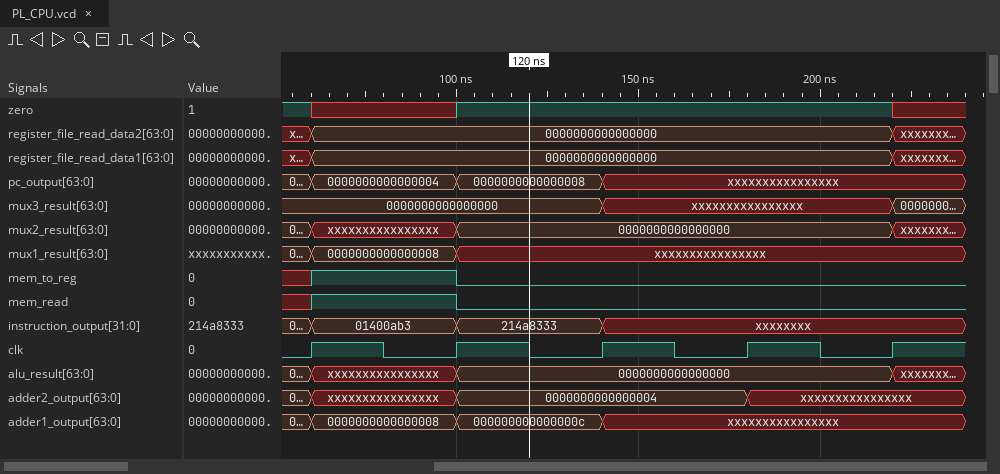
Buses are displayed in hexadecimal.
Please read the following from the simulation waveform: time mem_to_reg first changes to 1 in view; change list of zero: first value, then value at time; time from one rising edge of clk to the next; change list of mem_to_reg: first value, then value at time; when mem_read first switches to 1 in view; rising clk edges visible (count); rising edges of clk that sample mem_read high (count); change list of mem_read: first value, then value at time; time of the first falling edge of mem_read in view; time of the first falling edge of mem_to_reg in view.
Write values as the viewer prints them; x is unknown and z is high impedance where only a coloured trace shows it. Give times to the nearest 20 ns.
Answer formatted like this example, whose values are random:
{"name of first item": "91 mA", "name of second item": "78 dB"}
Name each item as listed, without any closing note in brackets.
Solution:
{"time mem_to_reg first changes to 1 in view": "60 ns", "change list of zero: first value, then value at time": "1, x at 60 ns, 1 at 100 ns, x at 220 ns", "time from one rising edge of clk to the next": "40 ns", "change list of mem_to_reg: first value, then value at time": "x, 1 at 60 ns, 0 at 100 ns", "when mem_read first switches to 1 in view": "60 ns", "rising clk edges visible": "5", "rising edges of clk that sample mem_read high": "1", "change list of mem_read: first value, then value at time": "x, 1 at 60 ns, 0 at 100 ns", "time of the first falling edge of mem_read in view": "100 ns", "time of the first falling edge of mem_to_reg in view": "100 ns"}
